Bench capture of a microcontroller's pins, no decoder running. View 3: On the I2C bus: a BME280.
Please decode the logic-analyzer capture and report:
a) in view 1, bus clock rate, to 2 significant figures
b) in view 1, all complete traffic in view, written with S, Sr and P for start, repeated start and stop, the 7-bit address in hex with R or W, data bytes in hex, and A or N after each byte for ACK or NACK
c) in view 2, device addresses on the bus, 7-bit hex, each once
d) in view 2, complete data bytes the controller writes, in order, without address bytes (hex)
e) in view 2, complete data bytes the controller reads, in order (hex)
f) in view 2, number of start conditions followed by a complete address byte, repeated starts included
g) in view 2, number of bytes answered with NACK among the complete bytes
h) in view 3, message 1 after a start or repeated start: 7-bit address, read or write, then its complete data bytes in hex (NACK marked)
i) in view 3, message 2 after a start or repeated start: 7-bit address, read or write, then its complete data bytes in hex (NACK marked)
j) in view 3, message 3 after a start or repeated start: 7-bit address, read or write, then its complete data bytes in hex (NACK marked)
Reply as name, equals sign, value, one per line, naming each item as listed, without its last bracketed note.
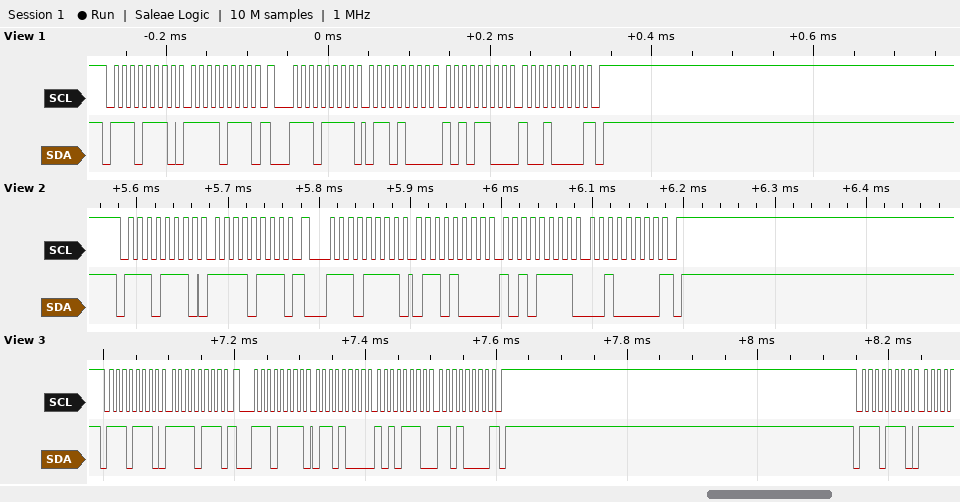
in view 1, bus clock rate, to 2 significant figures = 100 kHz
in view 1, all complete traffic in view, written with S, Sr and P for start, repeated start and stop, the 7-bit address in hex with R or W, data bytes in hex, and A or N after each byte for ACK or NACK = S 77W A F7 A Sr 77R A 68 A AC A 90 N P
in view 2, device addresses on the bus, 7-bit hex, each once = 0x77
in view 2, complete data bytes the controller writes, in order, without address bytes = F7
in view 2, complete data bytes the controller reads, in order = 68 AF 20
in view 2, number of start conditions followed by a complete address byte, repeated starts included = 2
in view 2, number of bytes answered with NACK among the complete bytes = 1
in view 3, message 1 after a start or repeated start: 7-bit address, read or write, then its complete data bytes in hex = 0x77 write: F7
in view 3, message 2 after a start or repeated start: 7-bit address, read or write, then its complete data bytes in hex = 0x77 read: 68 AE D0 NACK
in view 3, message 3 after a start or repeated start: 7-bit address, read or write, then its complete data bytes in hex = 0x77 write
